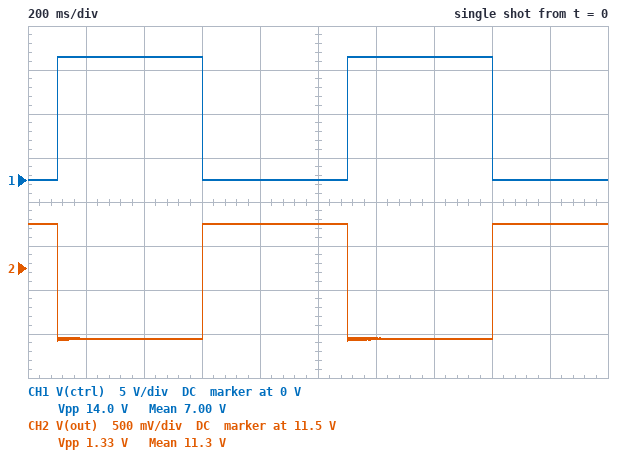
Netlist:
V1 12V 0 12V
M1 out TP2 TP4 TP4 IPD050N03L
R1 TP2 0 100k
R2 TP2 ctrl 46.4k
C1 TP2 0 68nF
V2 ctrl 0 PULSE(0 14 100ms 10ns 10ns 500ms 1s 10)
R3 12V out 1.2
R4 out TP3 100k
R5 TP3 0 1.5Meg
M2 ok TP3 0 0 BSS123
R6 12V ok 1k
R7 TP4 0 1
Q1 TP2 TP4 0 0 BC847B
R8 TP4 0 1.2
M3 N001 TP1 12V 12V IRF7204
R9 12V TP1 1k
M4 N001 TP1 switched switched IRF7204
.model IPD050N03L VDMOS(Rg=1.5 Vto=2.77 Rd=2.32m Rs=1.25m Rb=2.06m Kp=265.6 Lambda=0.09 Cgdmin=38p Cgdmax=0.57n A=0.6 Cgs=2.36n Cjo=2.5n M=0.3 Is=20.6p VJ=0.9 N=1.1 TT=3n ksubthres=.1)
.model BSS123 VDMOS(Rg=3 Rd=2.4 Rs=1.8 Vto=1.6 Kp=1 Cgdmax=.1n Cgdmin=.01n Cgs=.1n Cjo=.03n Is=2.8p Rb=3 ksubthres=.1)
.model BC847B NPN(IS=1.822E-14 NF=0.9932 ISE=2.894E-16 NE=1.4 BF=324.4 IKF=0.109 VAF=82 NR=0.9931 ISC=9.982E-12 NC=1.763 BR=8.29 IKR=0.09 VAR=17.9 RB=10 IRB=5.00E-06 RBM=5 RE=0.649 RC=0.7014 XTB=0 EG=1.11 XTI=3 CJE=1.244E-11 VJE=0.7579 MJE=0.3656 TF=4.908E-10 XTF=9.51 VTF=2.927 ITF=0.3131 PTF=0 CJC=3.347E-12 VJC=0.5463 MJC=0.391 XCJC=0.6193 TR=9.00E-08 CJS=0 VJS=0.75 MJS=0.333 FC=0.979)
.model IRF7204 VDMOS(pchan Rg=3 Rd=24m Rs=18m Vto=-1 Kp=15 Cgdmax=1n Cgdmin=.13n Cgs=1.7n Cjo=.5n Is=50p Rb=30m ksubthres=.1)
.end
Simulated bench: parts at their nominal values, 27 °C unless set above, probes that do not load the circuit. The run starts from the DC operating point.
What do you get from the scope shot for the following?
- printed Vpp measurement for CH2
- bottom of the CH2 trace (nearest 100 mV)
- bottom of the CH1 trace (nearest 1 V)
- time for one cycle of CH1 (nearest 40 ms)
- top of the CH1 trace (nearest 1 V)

1.33 V
10.7 V
0 V
1.00 s
14 V
